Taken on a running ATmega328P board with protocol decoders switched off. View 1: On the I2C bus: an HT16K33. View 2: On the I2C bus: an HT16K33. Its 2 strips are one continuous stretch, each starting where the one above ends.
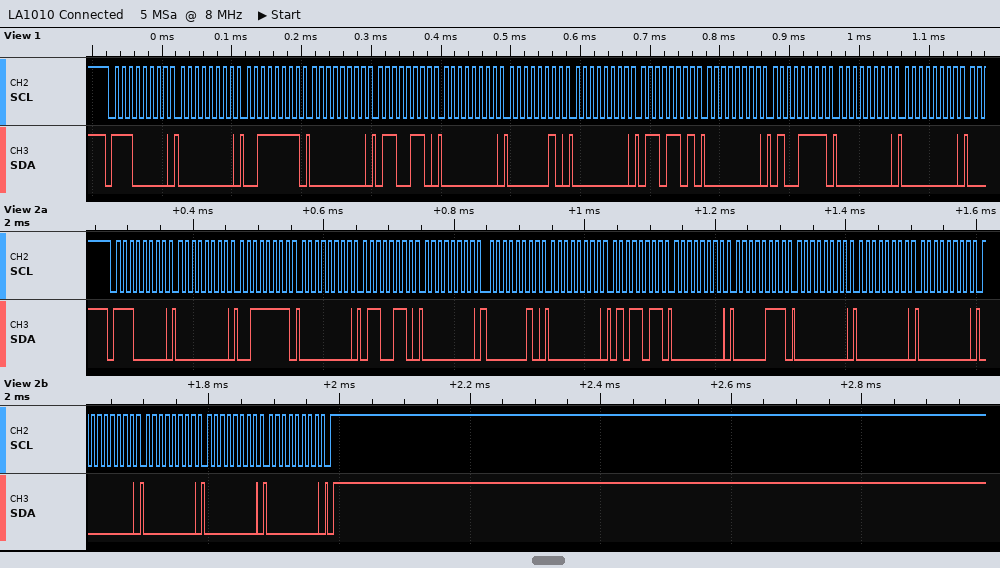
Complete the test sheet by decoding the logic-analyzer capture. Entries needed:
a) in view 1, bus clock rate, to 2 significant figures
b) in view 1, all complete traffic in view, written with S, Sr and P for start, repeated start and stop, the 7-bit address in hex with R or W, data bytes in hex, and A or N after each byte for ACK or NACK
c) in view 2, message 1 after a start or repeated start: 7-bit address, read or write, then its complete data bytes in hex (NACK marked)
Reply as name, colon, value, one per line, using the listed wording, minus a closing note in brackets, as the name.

in view 1, bus clock rate, to 2 significant figures: 100 kHz
in view 1, all complete traffic in view, written with S, Sr and P for start, repeated start and stop, the 7-bit address in hex with R or W, data bytes in hex, and A or N after each byte for ACK or NACK: S 70W A 00 A 3F A 00 A 66 A 00 A 02 A 00 A 6D A 00 A 4F A 00 A 00 A
in view 2, message 1 after a start or repeated start: 7-bit address, read or write, then its complete data bytes in hex: 0x70 write: 00 3F 00 66 00 02 00 5B 00 07 00 00 00 00 00 00 00
